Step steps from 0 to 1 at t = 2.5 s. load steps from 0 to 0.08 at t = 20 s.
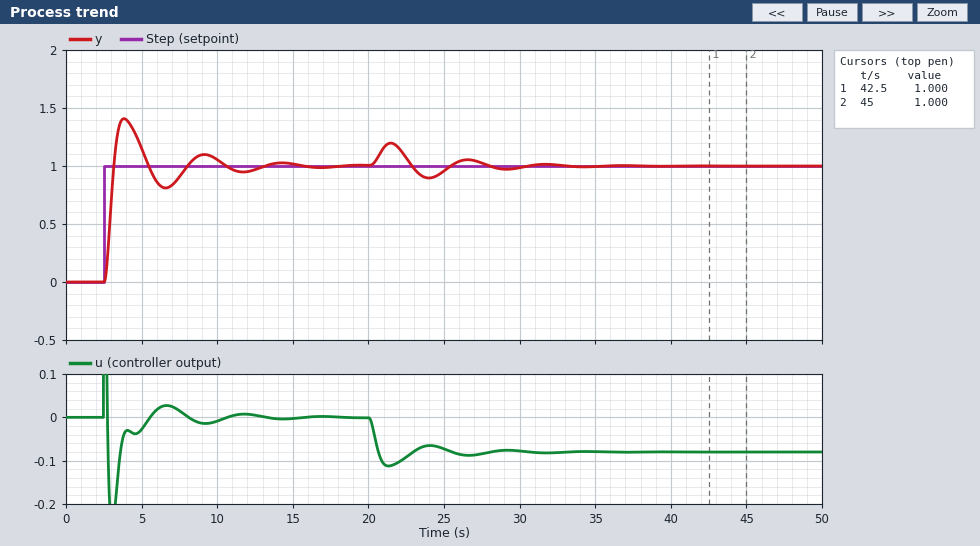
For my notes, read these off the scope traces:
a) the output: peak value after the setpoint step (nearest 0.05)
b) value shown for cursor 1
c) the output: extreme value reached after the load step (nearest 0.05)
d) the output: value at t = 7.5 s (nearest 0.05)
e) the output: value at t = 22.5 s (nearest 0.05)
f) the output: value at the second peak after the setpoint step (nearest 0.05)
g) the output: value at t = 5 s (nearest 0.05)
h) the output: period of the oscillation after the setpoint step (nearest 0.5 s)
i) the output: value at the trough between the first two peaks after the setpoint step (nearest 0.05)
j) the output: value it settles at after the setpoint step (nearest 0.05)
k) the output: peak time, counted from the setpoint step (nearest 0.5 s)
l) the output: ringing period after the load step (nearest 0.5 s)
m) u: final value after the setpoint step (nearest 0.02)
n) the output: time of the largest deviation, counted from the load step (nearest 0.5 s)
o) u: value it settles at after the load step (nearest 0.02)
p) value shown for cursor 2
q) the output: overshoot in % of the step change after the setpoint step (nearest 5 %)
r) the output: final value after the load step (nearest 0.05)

1.40
1.000
1.20
0.90
1.05
1.10
1.15
5.5 s
0.80
1.00
1.5 s
5.0 s
0.00
1.5 s
-0.08
1.000
40 %
1.00
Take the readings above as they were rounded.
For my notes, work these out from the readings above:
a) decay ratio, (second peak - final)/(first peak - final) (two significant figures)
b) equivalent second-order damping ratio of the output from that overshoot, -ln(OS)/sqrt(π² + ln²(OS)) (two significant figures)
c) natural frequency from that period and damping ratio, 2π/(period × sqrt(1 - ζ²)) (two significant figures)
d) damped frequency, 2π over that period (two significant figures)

0.25
0.28
1.2 rad/s
1.1 rad/s
